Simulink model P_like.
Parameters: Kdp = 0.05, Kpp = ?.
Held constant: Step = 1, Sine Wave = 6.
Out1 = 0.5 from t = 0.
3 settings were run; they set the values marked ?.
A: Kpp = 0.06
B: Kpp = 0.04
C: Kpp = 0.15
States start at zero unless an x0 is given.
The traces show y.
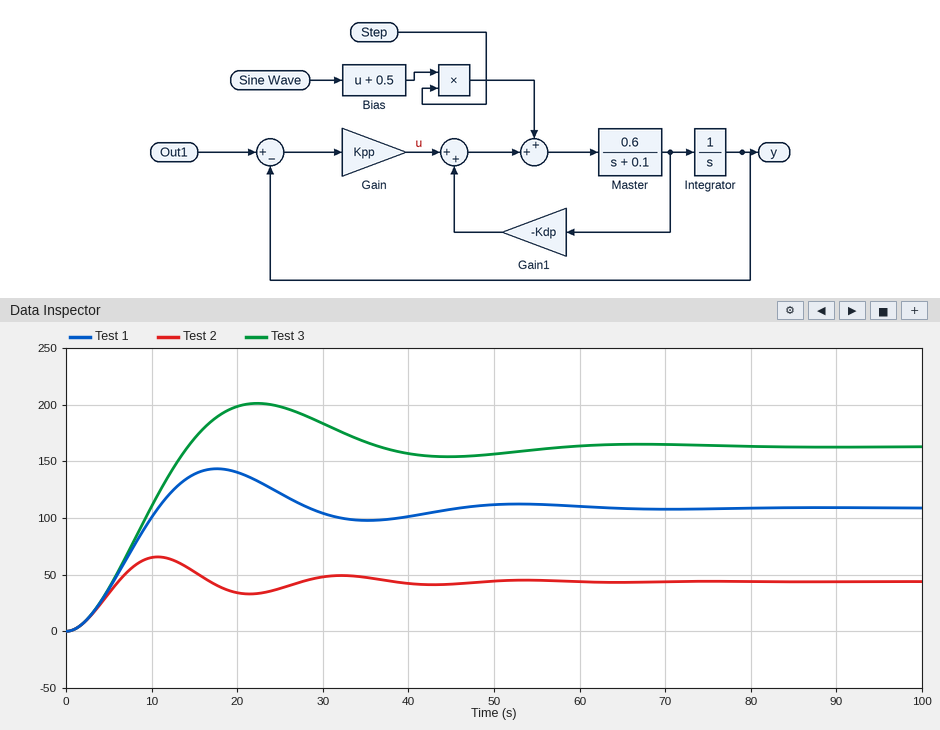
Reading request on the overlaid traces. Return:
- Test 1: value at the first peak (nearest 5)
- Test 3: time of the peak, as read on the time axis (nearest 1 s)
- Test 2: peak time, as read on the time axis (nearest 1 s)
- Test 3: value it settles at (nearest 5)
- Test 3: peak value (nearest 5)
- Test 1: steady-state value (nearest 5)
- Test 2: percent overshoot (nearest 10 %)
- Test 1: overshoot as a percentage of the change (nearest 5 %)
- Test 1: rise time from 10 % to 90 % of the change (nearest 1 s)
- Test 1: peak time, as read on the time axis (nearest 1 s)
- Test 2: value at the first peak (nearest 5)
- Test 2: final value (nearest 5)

145
22 s
11 s
165
200
110
50 %
30 %
7 s
18 s
65
45
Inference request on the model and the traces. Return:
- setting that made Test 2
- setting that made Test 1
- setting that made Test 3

C
A
B
